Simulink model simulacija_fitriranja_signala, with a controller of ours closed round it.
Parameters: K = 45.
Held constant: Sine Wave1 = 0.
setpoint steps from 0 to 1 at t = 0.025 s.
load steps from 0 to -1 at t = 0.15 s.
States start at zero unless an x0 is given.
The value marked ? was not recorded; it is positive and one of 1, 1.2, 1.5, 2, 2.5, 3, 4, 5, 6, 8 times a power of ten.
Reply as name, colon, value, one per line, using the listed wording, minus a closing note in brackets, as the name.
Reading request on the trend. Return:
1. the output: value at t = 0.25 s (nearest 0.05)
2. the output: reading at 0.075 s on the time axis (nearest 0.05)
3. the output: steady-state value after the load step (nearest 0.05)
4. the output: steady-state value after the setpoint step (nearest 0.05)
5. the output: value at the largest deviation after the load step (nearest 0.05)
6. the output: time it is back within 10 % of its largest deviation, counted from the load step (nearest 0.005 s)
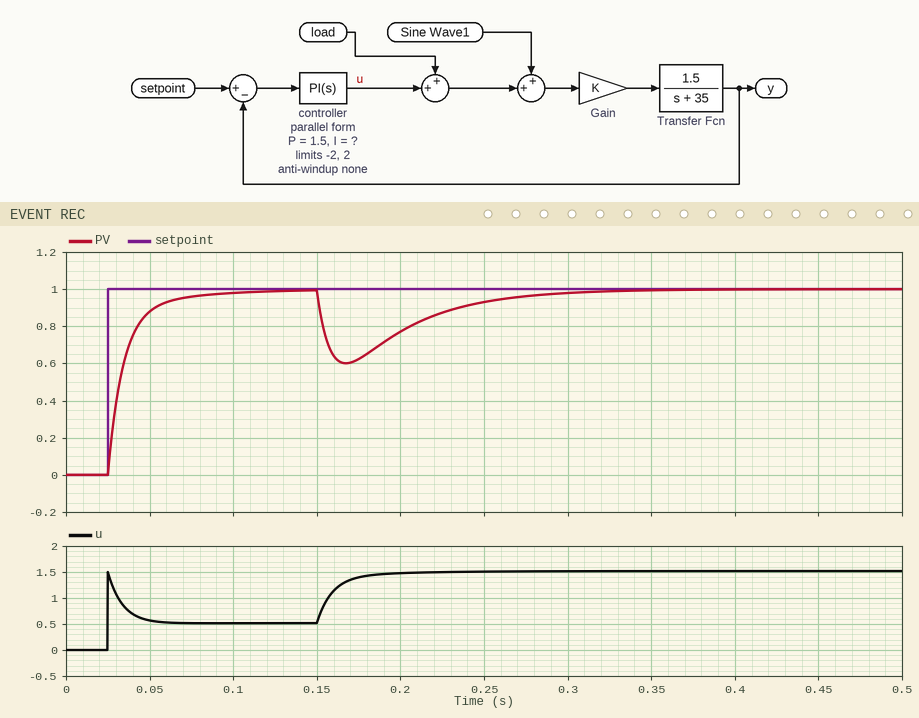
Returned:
the output: value at t = 0.25 s: 0.95
the output: reading at 0.075 s on the time axis: 0.95
the output: steady-state value after the load step: 1.00
the output: steady-state value after the setpoint step: 1.00
the output: value at the largest deviation after the load step: 0.60
the output: time it is back within 10 % of its largest deviation, counted from the load step: 0.125 s
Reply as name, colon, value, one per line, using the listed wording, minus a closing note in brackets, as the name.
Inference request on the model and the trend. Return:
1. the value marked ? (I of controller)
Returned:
the value marked ?: 40
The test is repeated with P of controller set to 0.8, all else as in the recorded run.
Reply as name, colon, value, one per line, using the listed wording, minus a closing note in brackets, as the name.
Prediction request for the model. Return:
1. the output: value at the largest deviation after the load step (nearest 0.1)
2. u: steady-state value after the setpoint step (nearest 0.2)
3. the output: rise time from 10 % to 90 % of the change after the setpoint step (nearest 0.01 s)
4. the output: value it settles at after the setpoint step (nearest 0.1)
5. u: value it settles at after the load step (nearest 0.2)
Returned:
the output: value at the largest deviation after the load step: 0.5
u: steady-state value after the setpoint step: 0.6
the output: rise time from 10 % to 90 % of the change after the setpoint step: 0.03 s
the output: value it settles at after the setpoint step: 1.0
u: value it settles at after the load step: 1.6
